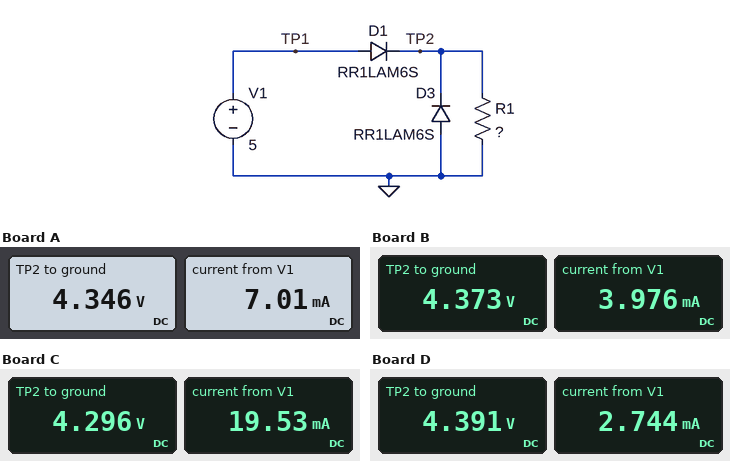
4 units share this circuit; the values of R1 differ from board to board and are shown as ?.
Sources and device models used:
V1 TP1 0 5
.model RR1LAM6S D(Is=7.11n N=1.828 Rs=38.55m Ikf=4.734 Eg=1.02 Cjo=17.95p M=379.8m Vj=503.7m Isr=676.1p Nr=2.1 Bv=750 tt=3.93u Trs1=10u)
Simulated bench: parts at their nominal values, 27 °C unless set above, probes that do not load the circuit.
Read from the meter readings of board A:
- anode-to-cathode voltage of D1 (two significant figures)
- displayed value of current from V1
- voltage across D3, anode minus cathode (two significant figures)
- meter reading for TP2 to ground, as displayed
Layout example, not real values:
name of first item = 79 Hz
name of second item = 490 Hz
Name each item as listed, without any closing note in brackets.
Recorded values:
anode-to-cathode voltage of D1 = 650 mV
displayed value of current from V1 = 7.01 mA
voltage across D3, anode minus cathode = -4.3 V
meter reading for TP2 to ground, as displayed = 4.346 V
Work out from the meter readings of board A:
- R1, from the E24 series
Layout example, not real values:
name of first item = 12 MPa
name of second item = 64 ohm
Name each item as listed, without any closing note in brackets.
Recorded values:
R1, from the E24 series = 620 Ω
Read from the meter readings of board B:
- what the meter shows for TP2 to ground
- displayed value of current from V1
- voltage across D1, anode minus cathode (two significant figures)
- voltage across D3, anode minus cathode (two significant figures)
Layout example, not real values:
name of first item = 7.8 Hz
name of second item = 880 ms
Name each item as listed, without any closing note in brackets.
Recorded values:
what the meter shows for TP2 to ground = 4.373 V
displayed value of current from V1 = 3.976 mA
voltage across D1, anode minus cathode = 630 mV
voltage across D3, anode minus cathode = -4.4 V
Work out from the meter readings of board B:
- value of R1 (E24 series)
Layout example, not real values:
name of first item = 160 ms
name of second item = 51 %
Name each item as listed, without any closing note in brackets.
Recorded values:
value of R1 = 1.1 kΩ
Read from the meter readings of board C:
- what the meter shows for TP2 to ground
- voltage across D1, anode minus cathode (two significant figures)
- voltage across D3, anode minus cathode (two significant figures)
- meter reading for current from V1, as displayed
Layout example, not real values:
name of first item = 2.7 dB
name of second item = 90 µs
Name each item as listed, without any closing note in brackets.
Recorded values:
what the meter shows for TP2 to ground = 4.296 V
voltage across D1, anode minus cathode = 700 mV
voltage across D3, anode minus cathode = -4.3 V
meter reading for current from V1, as displayed = 19.53 mA
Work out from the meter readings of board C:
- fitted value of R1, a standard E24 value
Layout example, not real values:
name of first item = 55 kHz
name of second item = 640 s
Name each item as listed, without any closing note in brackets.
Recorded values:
fitted value of R1, a standard E24 value = 220 Ω
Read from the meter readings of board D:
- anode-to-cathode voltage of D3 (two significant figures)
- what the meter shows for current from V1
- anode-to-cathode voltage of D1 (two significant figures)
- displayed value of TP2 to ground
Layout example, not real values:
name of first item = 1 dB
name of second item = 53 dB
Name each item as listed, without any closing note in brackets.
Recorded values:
anode-to-cathode voltage of D3 = -4.4 V
what the meter shows for current from V1 = 2.744 mA
anode-to-cathode voltage of D1 = 610 mV
displayed value of TP2 to ground = 4.391 V
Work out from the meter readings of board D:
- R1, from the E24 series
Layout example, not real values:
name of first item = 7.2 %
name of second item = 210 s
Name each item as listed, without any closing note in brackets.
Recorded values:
R1, from the E24 series = 1.6 kΩ
